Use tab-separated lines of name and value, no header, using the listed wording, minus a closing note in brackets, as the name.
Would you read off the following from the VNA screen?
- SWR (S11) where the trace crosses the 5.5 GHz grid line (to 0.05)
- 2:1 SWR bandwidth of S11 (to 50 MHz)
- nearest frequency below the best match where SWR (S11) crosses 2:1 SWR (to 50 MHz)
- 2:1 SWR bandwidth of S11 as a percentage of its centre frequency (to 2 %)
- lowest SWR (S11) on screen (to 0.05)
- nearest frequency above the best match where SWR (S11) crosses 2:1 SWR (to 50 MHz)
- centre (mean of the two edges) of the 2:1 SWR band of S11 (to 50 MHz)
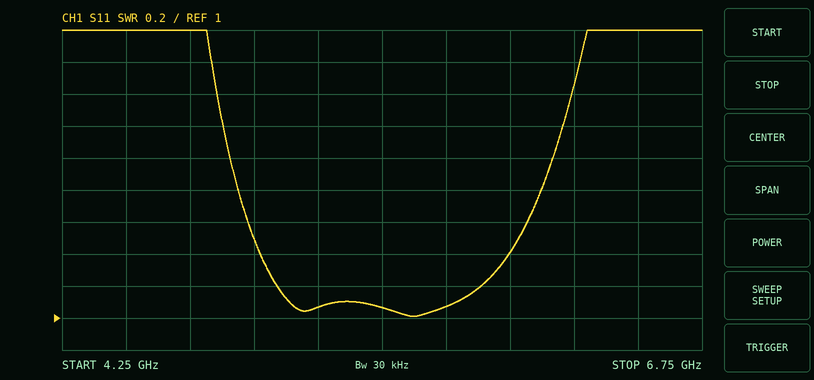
SWR (S11) where the trace crosses the 5.5 GHz grid line	1.05
2:1 SWR bandwidth of S11	1.25 GHz
nearest frequency below the best match where SWR (S11) crosses 2:1 SWR	4.90 GHz
2:1 SWR bandwidth of S11 as a percentage of its centre frequency	22 %
lowest SWR (S11) on screen	1.00
nearest frequency above the best match where SWR (S11) crosses 2:1 SWR	6.15 GHz
centre (mean of the two edges) of the 2:1 SWR band of S11	5.55 GHz
